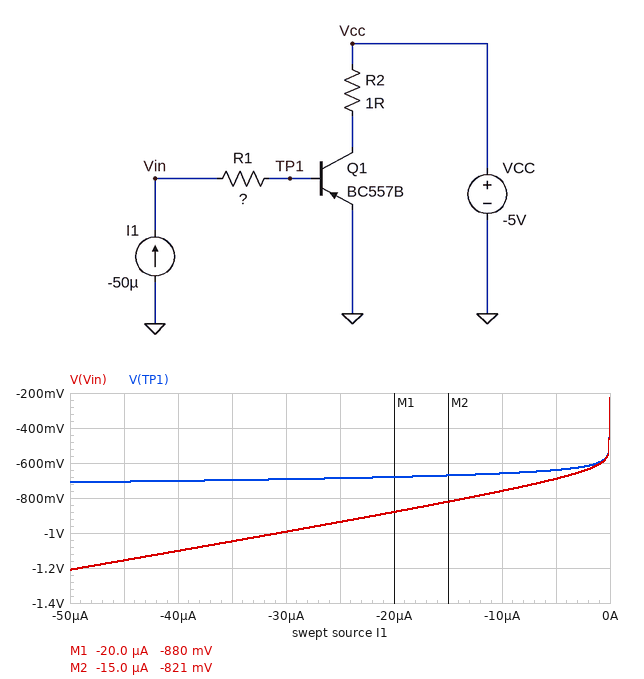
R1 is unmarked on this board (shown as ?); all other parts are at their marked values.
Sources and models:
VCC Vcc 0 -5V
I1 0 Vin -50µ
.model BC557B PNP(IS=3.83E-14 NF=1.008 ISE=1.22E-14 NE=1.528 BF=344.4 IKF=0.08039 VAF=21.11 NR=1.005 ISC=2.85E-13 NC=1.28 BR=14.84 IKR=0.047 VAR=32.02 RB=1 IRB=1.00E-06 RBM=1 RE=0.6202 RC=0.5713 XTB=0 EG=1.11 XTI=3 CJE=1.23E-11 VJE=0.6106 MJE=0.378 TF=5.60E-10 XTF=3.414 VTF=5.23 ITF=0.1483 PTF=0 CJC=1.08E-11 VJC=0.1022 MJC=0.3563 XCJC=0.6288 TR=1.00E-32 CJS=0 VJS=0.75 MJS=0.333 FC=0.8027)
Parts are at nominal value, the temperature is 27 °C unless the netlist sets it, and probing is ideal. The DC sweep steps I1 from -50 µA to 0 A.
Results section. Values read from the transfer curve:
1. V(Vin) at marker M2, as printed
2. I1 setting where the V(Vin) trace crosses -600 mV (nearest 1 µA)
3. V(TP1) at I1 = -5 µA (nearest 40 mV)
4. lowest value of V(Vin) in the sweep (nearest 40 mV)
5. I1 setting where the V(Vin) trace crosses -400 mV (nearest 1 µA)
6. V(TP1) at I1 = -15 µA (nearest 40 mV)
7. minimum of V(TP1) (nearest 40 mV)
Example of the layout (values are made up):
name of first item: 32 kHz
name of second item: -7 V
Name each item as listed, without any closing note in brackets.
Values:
V(Vin) at marker M2, as printed: -821 mV
I1 setting where the V(Vin) trace crosses -600 mV: -1 µA
V(TP1) at I1 = -5 µA: -640 mV
lowest value of V(Vin) in the sweep: -1.20 V
I1 setting where the V(Vin) trace crosses -400 mV: 0 A
V(TP1) at I1 = -15 µA: -680 mV
minimum of V(TP1): -720 mV
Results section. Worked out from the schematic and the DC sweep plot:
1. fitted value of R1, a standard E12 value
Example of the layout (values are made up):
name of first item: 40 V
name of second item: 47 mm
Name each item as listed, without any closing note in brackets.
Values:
fitted value of R1, a standard E12 value: 10 kΩ
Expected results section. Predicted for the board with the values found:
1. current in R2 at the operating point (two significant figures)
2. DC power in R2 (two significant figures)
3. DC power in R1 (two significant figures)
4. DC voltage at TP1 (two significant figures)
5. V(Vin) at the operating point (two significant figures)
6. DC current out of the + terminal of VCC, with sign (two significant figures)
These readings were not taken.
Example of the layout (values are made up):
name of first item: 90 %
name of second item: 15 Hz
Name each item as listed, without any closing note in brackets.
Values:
current in R2 at the operating point: 17 mA
DC power in R2: 290 µW
DC power in R1: 25 µW
DC voltage at TP1: -710 mV
V(Vin) at the operating point: -1.2 V
DC current out of the + terminal of VCC, with sign: -17 mA
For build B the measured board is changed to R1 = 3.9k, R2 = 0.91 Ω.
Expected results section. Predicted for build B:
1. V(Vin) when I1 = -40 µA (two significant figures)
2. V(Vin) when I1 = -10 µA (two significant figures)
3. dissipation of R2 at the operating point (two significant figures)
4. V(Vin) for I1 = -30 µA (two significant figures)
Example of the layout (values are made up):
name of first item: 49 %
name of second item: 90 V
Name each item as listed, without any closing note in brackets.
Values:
V(Vin) when I1 = -40 µA: -860 mV
V(Vin) when I1 = -10 µA: -700 mV
dissipation of R2 at the operating point: 260 µW
V(Vin) for I1 = -30 µA: -810 mV
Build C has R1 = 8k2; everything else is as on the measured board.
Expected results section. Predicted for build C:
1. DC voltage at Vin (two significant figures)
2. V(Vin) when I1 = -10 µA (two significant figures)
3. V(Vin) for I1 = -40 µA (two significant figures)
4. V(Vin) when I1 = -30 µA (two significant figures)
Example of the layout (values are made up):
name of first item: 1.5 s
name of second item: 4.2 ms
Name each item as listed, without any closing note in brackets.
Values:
DC voltage at Vin: -1.1 V
V(Vin) when I1 = -10 µA: -740 mV
V(Vin) for I1 = -40 µA: -1.0 V
V(Vin) when I1 = -30 µA: -940 mV
